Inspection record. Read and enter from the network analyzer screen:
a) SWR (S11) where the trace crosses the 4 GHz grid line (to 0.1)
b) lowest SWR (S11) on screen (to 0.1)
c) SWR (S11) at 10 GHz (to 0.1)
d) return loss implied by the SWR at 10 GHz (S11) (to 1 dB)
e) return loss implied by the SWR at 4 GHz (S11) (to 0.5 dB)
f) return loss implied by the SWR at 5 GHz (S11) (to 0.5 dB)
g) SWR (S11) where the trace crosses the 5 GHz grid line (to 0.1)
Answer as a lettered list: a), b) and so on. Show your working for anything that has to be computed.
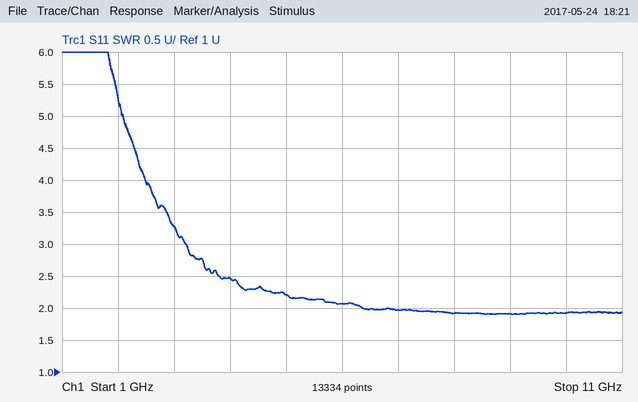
a) 2.5
b) 1.9
c) 1.9
d) −20 log10((1.9 − 1)/(1.9 + 1)) ≈ 10 dB
e) −20 log10((2.5 − 1)/(2.5 + 1)) ≈ 7.36 dB, so 7.5 dB to the nearest 0.5 dB
f) −20 log10((2.2 − 1)/(2.2 + 1)) ≈ 8.5 dB
g) 2.2
